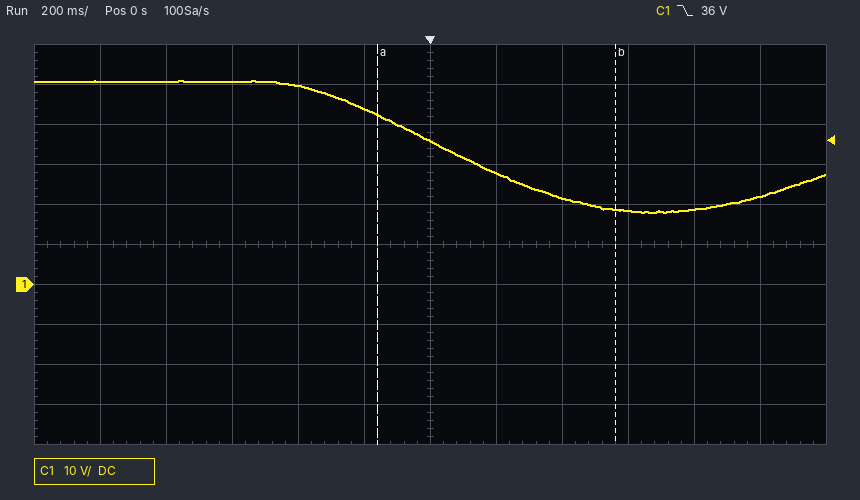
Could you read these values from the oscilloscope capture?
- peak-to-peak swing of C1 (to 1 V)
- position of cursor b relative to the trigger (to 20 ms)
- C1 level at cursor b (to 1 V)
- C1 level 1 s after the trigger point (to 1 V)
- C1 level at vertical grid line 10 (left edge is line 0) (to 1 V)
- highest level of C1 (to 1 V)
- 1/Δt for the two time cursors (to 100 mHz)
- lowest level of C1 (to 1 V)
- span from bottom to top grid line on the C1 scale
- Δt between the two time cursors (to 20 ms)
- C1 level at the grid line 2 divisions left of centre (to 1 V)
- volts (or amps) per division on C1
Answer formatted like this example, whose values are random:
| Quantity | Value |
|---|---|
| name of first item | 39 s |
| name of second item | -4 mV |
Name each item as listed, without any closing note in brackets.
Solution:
| Quantity | Value |
|---|---|
| peak-to-peak swing of C1 | 33 V |
| position of cursor b relative to the trigger | +560 ms |
| C1 level at cursor b | 19 V |
| C1 level 1 s after the trigger point | 22 V |
| C1 level at vertical grid line 10 (left edge is line 0) | 19 V |
| highest level of C1 | 51 V |
| 1/Δt for the two time cursors | 1.4 Hz |
| lowest level of C1 | 18 V |
| span from bottom to top grid line on the C1 scale | 100 V |
| Δt between the two time cursors | 720 ms |
| C1 level at the grid line 2 divisions left of centre | 50 V |
| volts (or amps) per division on C1 | 10 V |
